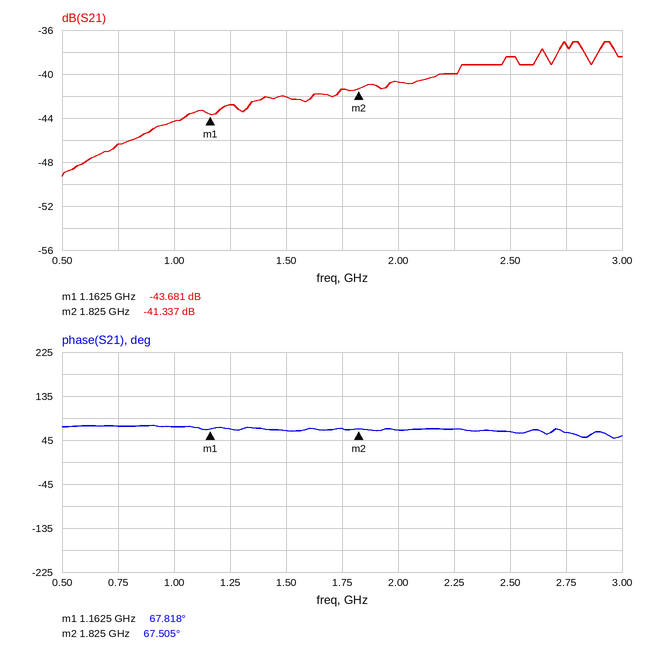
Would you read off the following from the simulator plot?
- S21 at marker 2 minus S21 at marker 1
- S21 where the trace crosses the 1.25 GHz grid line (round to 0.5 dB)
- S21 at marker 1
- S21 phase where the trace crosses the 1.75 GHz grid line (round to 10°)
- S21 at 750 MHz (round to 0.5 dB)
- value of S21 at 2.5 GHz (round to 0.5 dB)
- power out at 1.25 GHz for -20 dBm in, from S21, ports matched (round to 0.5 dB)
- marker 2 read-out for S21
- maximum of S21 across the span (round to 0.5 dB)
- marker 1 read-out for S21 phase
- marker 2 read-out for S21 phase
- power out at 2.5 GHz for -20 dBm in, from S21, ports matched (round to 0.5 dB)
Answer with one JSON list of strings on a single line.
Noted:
["2.344 dB", "-43.0 dB", "-43.681 dB", "70°", "-46.5 dB", "-38.5 dB", "-63.0 dBm", "-41.337 dB", "-37.0 dB", "67.818°", "67.505°", "-58.5 dBm"]
